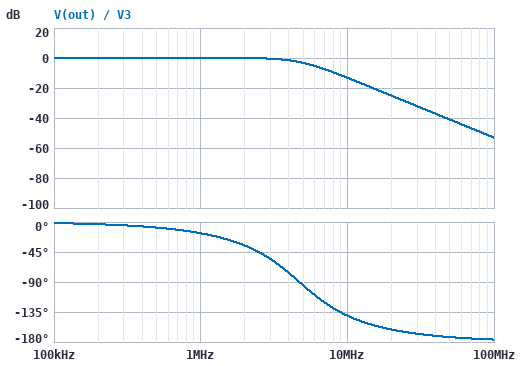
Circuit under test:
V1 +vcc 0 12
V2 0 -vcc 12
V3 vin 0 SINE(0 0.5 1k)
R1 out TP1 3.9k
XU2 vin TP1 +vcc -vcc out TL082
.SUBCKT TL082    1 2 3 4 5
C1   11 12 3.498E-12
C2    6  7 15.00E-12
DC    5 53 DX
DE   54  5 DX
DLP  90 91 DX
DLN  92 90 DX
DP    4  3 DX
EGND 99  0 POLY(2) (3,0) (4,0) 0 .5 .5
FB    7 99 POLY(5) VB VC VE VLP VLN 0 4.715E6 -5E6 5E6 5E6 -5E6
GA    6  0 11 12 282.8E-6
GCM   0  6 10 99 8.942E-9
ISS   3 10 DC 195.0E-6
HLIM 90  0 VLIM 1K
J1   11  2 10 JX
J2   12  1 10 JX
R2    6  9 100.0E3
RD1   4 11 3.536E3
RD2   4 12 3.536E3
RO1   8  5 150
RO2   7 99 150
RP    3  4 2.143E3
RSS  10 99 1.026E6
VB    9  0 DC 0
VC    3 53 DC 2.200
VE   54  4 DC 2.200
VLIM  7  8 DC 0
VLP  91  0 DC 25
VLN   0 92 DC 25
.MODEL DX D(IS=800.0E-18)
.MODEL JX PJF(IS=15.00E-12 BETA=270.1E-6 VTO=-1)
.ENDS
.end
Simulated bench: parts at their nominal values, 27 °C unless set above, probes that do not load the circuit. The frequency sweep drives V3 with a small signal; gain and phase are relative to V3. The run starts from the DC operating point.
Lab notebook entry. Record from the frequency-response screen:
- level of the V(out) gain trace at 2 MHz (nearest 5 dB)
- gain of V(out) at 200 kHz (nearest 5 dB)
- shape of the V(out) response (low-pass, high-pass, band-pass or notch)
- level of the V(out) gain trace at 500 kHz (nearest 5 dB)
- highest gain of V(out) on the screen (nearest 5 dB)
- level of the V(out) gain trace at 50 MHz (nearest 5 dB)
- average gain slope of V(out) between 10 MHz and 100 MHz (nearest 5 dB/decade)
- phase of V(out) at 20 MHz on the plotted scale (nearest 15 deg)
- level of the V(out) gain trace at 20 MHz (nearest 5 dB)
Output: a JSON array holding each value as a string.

["0 dB", "0 dB", "low-pass", "0 dB", "0 dB", "-40 dB", "-40 dB/decade", "-165 deg", "-25 dB"]
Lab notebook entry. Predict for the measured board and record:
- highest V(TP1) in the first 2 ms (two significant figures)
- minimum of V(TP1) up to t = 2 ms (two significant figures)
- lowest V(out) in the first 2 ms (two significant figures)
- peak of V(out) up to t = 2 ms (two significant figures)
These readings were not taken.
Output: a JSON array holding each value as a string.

["500 mV", "-500 mV", "-500 mV", "500 mV"]
